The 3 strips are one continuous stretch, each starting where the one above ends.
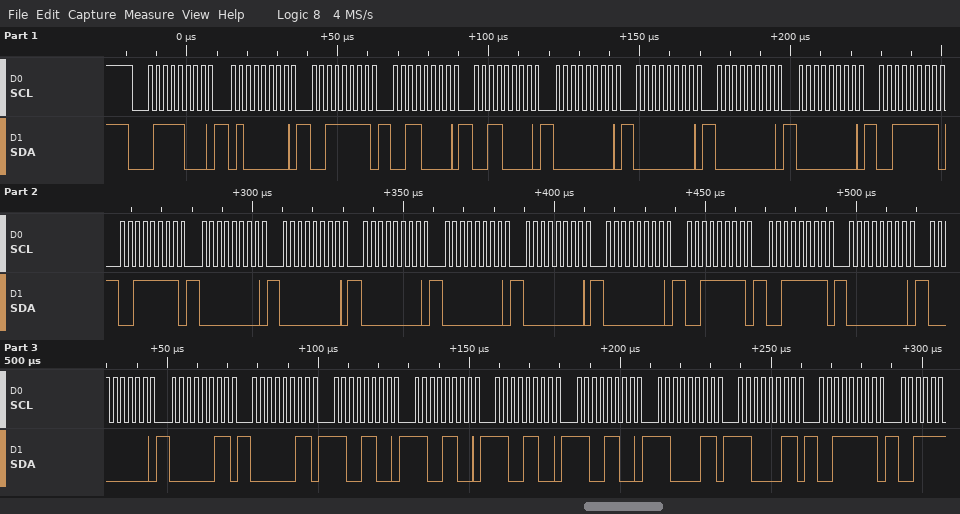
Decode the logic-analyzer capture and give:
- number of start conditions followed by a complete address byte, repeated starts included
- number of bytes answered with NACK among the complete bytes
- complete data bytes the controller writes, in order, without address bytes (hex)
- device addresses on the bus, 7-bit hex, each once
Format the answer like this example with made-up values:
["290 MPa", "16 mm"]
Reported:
["1", "0", "40 3F 30 30 00 00 00 00 3F 3F 00 00 00 00 00 00 3F 3F 00 00 03 03 CC CC CC CC C3 C3 3F", "0x3C"]
